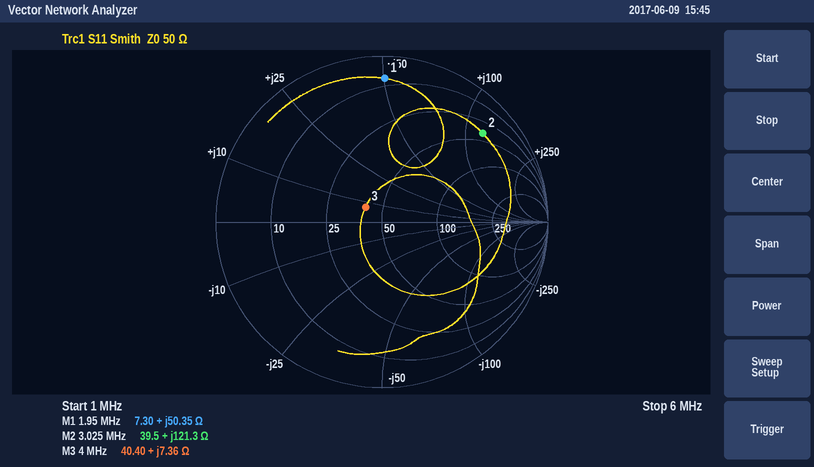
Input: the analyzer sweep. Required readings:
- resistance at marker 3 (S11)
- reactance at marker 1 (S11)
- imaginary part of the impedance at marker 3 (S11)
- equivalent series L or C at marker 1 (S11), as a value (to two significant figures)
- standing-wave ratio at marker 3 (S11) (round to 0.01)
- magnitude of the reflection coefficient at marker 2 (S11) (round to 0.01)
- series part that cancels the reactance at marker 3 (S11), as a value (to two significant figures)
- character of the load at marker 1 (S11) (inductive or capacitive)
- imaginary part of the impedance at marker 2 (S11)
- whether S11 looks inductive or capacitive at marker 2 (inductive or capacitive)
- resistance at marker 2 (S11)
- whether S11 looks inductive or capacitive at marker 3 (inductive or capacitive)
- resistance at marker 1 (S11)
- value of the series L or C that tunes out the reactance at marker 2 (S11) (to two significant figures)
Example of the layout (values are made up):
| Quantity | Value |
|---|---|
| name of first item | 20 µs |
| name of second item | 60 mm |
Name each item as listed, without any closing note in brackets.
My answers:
| Quantity | Value |
|---|---|
| resistance at marker 3 | 40.40 Ω |
| reactance at marker 1 | +50.35 Ω |
| imaginary part of the impedance at marker 3 | +7.36 Ω |
| equivalent series L or C at marker 1 (S11), as a value | 4.1 µH |
| standing-wave ratio at marker 3 (S11) | 1.31 |
| magnitude of the reflection coefficient at marker 2 (S11) | 0.81 |
| series part that cancels the reactance at marker 3 (S11), as a value | 5.4 nF |
| character of the load at marker 1 (S11) | inductive |
| imaginary part of the impedance at marker 2 | +121.3 Ω |
| whether S11 looks inductive or capacitive at marker 2 | inductive |
| resistance at marker 2 | 39.5 Ω |
| whether S11 looks inductive or capacitive at marker 3 | inductive |
| resistance at marker 1 | 7.30 Ω |
| value of the series L or C that tunes out the reactance at marker 2 (S11) | 430 pF |
